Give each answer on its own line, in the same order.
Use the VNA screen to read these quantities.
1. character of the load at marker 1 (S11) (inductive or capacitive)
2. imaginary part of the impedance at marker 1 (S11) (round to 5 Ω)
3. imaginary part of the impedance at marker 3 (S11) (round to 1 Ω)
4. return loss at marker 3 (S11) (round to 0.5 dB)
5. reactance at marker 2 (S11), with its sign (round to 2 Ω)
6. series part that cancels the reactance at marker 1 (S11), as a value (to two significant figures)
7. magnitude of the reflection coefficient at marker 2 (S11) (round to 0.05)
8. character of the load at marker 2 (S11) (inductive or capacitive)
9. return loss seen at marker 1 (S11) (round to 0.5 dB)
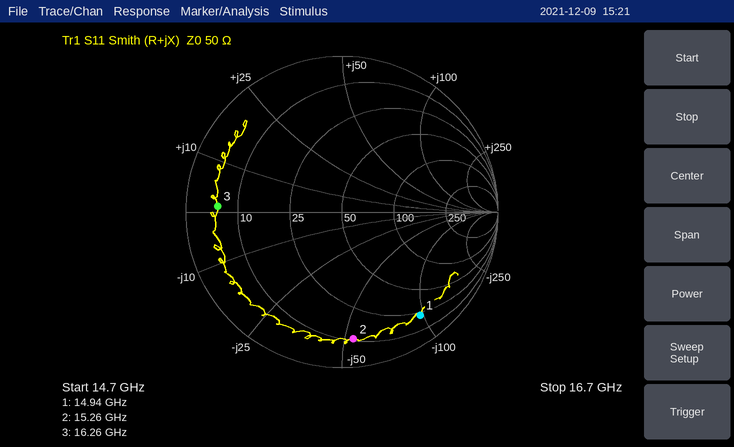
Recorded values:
capacitive
-95 Ω
+1 Ω
2.0 dB
-54 Ω
1.0 nH
0.80
capacitive
1.5 dB
